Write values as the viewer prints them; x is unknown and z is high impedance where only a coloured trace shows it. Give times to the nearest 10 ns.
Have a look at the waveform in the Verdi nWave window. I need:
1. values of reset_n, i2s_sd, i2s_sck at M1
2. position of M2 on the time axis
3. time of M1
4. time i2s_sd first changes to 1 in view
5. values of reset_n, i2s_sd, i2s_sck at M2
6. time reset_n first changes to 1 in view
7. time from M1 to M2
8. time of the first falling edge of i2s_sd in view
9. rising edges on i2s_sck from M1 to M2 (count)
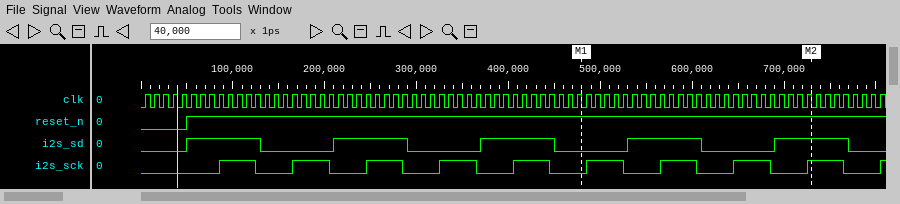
reset_n=1, i2s_sd=0, i2s_sck=0
730 ns
480 ns
50 ns
reset_n=1, i2s_sd=1, i2s_sck=1
50 ns
250 ns
130 ns
4
